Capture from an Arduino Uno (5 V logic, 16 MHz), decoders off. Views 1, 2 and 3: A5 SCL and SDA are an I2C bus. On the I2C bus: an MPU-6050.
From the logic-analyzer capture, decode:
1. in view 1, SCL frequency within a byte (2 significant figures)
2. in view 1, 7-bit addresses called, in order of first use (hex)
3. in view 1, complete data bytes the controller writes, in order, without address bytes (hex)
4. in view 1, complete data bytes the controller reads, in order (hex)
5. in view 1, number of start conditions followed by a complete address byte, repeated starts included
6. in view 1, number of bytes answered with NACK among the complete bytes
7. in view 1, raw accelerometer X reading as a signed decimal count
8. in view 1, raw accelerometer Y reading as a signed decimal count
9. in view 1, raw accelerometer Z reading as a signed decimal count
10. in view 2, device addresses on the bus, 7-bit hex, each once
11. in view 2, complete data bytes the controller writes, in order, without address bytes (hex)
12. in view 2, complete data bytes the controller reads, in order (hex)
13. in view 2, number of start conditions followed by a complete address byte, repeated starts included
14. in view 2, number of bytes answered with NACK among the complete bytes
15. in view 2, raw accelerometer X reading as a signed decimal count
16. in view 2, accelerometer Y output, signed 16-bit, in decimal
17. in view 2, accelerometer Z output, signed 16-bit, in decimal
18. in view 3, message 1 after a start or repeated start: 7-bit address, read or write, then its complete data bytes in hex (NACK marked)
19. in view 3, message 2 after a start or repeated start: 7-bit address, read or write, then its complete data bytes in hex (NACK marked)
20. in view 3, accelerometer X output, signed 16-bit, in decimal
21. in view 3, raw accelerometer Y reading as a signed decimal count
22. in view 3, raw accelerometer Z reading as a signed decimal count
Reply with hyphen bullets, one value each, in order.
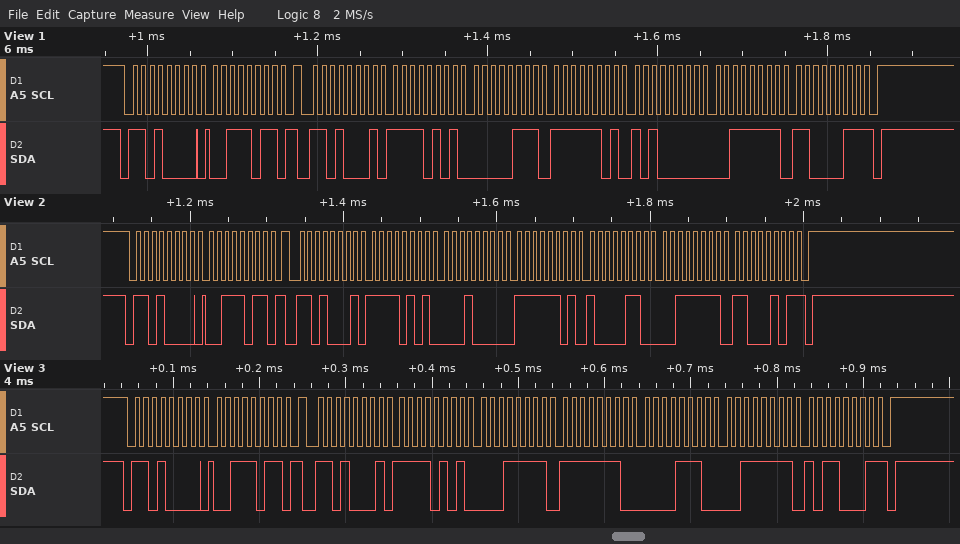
- 100 kHz
- 0x68
- 3B
- F5 07 FD A0 3F C3
- 2
- 1
- -2809
- -608
- 16323
- 0x68
- 3B
- F5 10 FD 86 3F C5
- 2
- 1
- -2800
- -634
- 16325
- 0x68 write: 3B
- 0x68 read: F5 1F FE 0E 3F B1 NACK
- -2785
- -498
- 16305
